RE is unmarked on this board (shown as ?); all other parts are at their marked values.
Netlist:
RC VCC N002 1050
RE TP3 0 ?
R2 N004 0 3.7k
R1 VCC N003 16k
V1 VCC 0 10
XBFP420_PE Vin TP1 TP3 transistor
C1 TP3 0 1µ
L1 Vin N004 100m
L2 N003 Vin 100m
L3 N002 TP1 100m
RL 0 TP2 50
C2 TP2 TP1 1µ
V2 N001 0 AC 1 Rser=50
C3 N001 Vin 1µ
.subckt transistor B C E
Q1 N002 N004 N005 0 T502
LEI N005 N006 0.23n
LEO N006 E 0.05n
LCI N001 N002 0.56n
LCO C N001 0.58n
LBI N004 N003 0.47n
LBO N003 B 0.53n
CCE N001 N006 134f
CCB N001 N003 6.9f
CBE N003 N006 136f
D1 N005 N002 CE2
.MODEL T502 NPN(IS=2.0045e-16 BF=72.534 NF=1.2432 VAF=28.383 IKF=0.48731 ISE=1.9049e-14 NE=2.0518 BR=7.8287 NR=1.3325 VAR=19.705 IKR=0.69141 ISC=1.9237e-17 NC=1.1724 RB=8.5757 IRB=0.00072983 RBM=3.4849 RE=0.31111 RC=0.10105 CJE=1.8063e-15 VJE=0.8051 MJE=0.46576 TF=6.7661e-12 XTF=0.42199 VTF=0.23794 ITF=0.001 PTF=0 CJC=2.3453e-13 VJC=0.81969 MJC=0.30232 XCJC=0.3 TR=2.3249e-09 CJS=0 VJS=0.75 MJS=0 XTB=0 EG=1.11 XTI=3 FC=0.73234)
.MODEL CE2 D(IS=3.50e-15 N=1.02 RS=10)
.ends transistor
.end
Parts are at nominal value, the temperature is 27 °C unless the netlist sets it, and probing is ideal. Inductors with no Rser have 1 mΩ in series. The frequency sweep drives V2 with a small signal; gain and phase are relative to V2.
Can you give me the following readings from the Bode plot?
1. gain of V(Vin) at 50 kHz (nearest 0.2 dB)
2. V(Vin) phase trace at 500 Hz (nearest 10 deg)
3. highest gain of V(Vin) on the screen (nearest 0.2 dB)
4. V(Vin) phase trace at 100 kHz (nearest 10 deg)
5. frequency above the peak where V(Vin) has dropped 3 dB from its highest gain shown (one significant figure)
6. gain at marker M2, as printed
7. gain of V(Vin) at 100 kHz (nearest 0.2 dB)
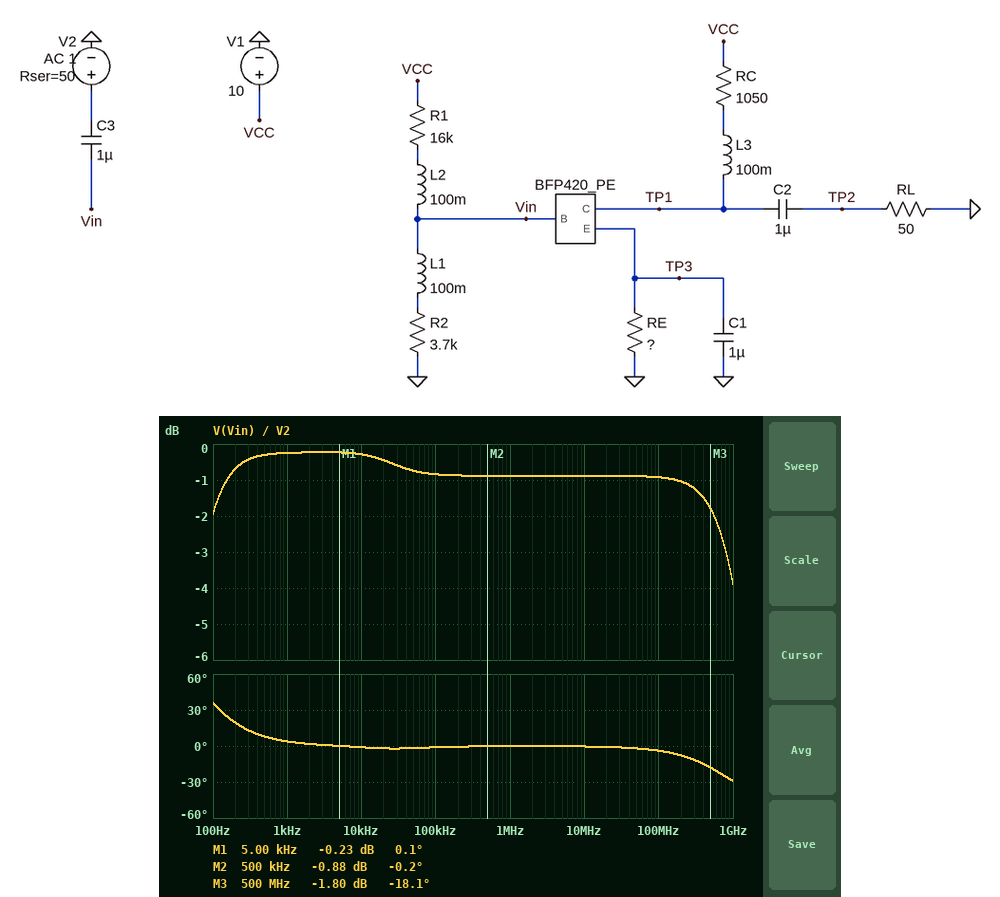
-0.8 dB
10 deg
-0.2 dB
0 deg
900 MHz
-0.88 dB
-0.8 dB
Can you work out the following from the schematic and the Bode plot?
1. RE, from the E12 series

120 Ω
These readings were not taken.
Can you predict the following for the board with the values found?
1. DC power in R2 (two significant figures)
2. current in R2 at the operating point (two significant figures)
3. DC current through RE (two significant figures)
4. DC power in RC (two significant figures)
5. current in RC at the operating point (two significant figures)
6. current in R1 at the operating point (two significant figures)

740 µW
450 µA
5.5 mA
31 mW
5.4 mA
520 µA
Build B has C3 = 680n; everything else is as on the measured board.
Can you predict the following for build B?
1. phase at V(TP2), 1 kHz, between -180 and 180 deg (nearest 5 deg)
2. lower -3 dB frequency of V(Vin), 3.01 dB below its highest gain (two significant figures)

-130 deg
100 Hz
